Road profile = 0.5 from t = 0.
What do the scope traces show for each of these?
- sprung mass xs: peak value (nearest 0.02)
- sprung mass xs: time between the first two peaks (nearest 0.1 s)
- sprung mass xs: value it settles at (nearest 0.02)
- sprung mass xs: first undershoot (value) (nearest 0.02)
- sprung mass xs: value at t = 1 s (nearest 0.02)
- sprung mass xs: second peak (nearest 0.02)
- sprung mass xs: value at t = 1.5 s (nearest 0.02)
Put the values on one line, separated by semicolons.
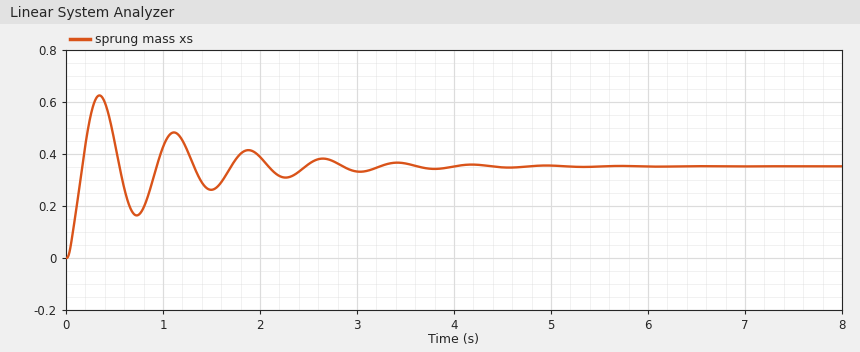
0.62; 0.8 s; 0.36; 0.16; 0.42; 0.48; 0.26
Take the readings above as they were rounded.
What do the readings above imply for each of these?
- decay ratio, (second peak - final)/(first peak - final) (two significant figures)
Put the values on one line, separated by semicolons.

0.46
